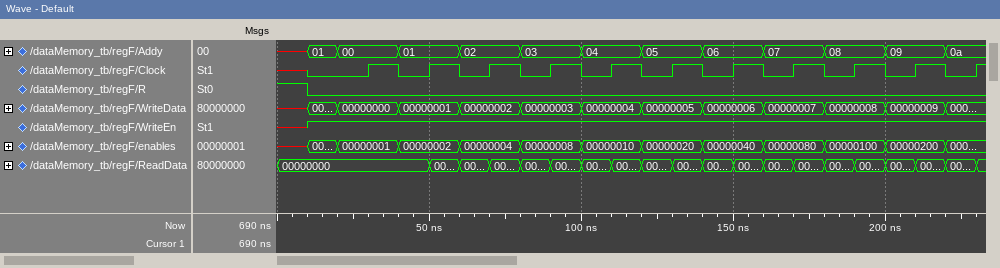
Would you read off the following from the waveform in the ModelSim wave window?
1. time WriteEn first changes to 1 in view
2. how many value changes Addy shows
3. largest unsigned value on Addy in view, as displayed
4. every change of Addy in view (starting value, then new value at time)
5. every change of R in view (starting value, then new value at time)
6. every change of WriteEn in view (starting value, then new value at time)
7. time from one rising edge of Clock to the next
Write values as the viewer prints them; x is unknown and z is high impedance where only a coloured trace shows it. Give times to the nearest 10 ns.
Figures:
10 ns
12
0a
x, 01 at 10 ns, 00 at 20 ns, 01 at 40 ns, 02 at 60 ns, 03 at 80 ns, 04 at 100 ns, 05 at 120 ns, 06 at 140 ns, 07 at 160 ns, 08 at 180 ns, 09 at 200 ns, 0a at 220 ns
1, 0 at 10 ns
x, 1 at 10 ns
20 ns
